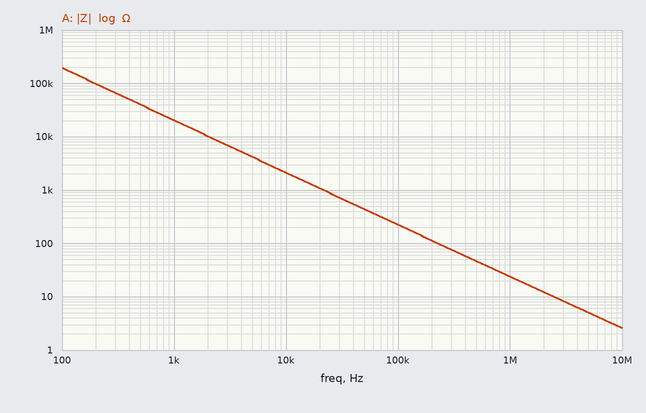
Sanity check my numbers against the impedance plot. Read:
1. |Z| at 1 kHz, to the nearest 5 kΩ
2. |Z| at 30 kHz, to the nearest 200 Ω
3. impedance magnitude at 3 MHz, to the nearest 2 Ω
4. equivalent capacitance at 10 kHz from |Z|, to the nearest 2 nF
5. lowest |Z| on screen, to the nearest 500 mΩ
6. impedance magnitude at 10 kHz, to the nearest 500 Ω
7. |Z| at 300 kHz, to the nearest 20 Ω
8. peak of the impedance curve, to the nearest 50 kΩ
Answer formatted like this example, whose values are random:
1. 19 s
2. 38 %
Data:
1. 20 kΩ
2. 800 Ω
3. 8 Ω
4. 8 nF
5. 2.5 Ω
6. 2.0 kΩ
7. 80 Ω
8. 200 kΩ
